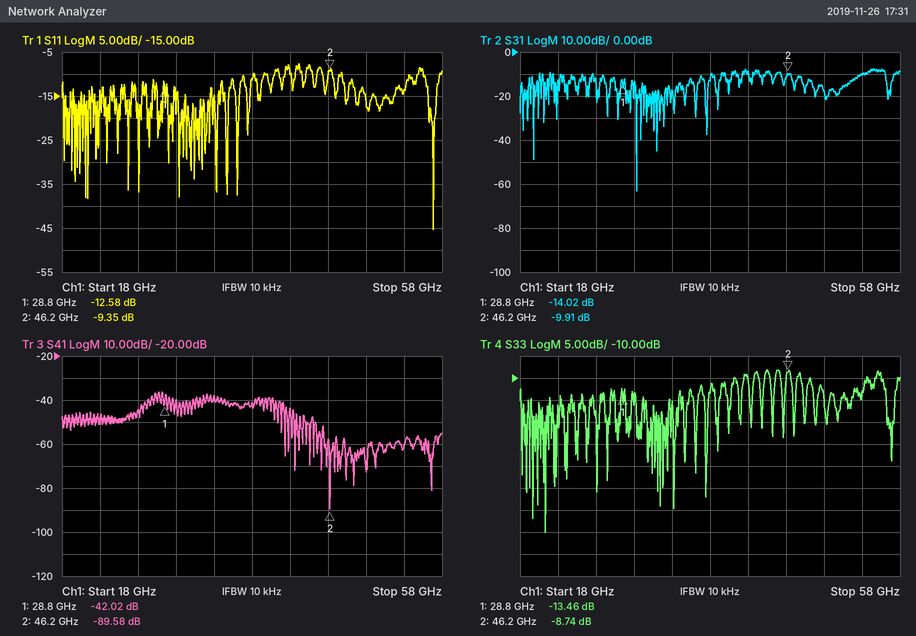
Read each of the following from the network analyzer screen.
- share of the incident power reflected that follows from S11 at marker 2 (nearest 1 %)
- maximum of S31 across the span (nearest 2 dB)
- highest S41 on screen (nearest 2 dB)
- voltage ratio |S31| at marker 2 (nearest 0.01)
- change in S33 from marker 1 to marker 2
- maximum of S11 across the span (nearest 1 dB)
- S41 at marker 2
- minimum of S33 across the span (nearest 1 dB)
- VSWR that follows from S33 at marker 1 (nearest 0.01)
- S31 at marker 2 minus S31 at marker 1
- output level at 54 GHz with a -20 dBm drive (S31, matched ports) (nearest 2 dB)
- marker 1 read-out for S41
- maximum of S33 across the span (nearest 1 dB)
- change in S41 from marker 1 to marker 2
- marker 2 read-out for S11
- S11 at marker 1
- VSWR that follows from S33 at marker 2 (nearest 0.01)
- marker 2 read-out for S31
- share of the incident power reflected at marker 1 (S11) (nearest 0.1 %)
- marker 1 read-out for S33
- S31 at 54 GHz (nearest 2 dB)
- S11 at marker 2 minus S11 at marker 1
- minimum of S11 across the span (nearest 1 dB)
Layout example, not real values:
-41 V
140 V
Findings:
12 %
-8 dB
-36 dB
0.32
4.72 dB
-8 dB
-89.58 dB
-45 dB
1.54
4.11 dB
-30 dBm
-42.02 dB
-8 dB
-47.56 dB
-9.35 dB
-12.58 dB
2.15
-9.91 dB
5.5 %
-13.46 dB
-10 dB
3.23 dB
-45 dB
